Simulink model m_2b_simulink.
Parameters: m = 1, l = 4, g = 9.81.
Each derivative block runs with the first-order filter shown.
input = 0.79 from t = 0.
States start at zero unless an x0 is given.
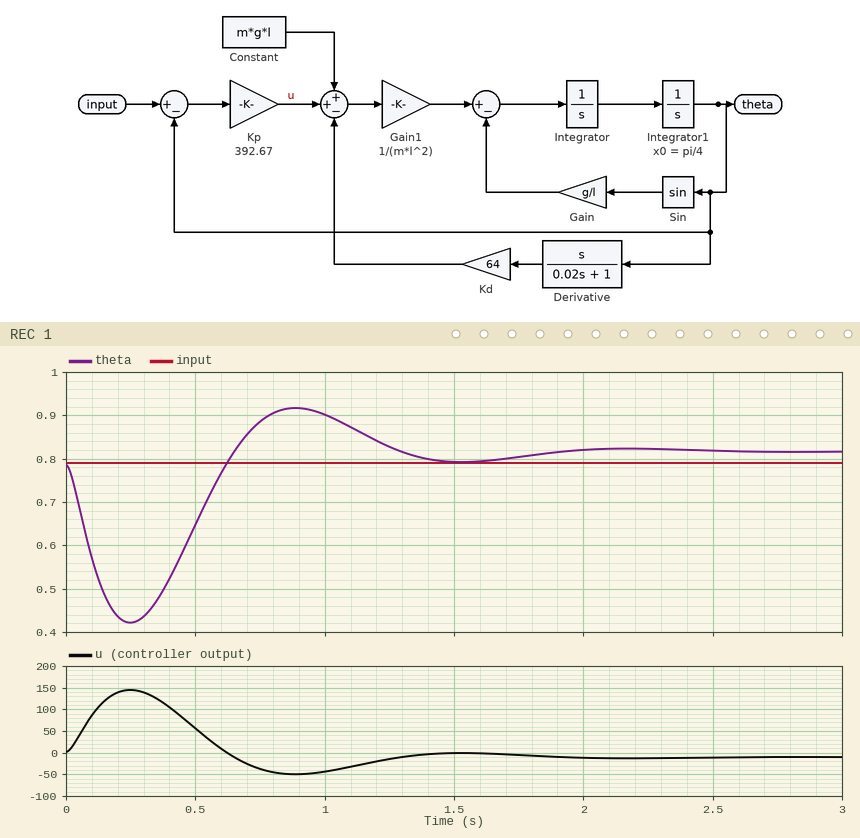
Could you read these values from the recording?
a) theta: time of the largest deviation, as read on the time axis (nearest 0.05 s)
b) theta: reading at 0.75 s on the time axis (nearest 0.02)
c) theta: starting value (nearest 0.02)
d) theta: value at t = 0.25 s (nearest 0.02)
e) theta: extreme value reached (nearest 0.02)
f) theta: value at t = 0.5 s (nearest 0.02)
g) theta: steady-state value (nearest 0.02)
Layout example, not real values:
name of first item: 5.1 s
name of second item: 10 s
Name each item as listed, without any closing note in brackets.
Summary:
theta: time of the largest deviation, as read on the time axis: 0.25 s
theta: reading at 0.75 s on the time axis: 0.88
theta: starting value: 0.78
theta: value at t = 0.25 s: 0.42
theta: extreme value reached: 0.42
theta: value at t = 0.5 s: 0.64
theta: steady-state value: 0.82
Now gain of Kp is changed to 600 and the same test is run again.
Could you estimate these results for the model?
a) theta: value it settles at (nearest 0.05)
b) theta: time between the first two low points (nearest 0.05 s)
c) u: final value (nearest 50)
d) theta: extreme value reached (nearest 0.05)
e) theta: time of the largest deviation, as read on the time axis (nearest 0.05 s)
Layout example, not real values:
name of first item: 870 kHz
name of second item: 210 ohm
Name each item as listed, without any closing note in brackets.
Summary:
theta: value it settles at: 0.80
theta: time between the first two low points: 1.00 s
u: final value: 0
theta: extreme value reached: 0.45
theta: time of the largest deviation, as read on the time axis: 0.20 s
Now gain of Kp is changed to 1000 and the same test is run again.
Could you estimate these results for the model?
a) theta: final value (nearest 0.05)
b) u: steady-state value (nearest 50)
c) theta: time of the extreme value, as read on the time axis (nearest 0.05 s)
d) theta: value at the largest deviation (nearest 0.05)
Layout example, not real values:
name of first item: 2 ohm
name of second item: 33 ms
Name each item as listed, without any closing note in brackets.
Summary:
theta: final value: 0.80
u: steady-state value: 0
theta: time of the extreme value, as read on the time axis: 0.20 s
theta: value at the largest deviation: 0.50
